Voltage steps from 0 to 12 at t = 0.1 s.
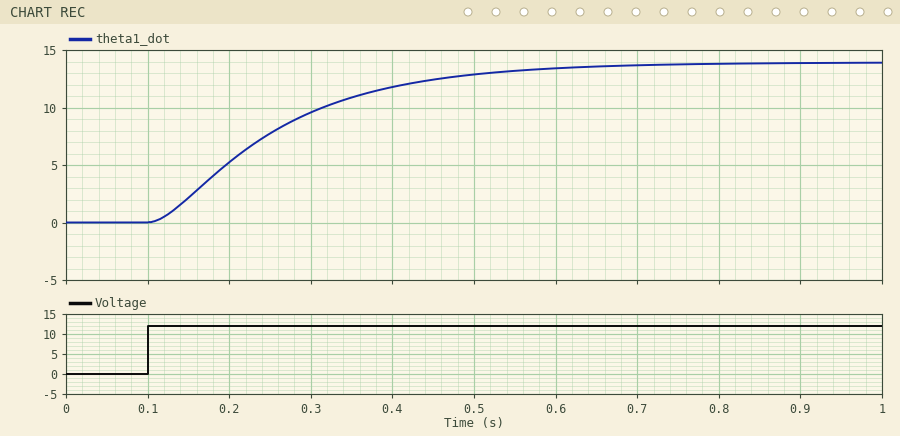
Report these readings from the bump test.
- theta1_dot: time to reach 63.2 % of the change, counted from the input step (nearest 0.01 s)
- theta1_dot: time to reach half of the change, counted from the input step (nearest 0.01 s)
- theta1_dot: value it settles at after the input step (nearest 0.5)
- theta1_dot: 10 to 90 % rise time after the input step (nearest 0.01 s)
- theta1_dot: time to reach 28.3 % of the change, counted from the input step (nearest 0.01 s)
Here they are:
0.18 s
0.13 s
14.0
0.32 s
0.08 s
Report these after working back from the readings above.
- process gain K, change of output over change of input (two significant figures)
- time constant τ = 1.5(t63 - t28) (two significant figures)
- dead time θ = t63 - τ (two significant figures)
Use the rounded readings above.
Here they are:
1.2
0.15 s
0.030 s
